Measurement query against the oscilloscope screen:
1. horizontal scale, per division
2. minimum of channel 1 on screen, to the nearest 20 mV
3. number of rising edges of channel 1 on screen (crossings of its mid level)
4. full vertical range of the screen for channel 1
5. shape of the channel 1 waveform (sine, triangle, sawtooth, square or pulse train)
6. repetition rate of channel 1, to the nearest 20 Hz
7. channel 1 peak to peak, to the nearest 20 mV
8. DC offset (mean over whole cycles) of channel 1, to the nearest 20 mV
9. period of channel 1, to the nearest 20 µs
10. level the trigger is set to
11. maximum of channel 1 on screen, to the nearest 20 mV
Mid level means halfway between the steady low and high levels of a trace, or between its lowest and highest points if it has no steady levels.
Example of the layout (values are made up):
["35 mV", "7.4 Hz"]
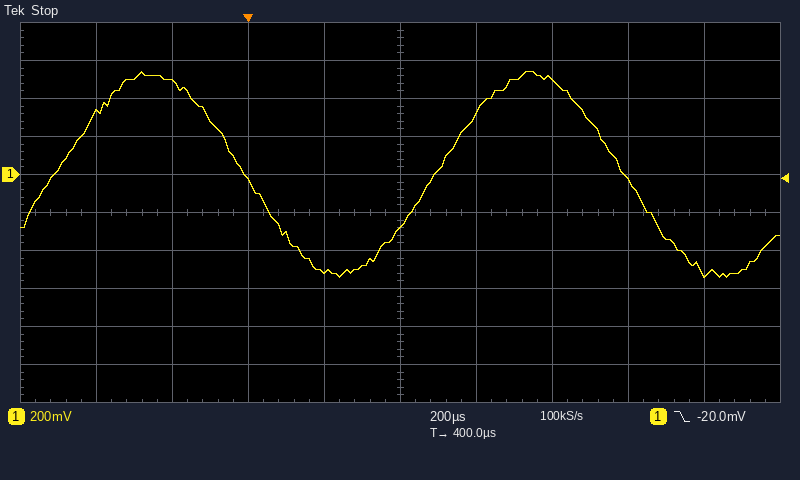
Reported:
["200 µs", "-540 mV", "2", "2 V", "sine", "1.00 kHz", "1.08 V", "0 mV", "1.00 ms", "-20.0 mV", "540 mV"]
